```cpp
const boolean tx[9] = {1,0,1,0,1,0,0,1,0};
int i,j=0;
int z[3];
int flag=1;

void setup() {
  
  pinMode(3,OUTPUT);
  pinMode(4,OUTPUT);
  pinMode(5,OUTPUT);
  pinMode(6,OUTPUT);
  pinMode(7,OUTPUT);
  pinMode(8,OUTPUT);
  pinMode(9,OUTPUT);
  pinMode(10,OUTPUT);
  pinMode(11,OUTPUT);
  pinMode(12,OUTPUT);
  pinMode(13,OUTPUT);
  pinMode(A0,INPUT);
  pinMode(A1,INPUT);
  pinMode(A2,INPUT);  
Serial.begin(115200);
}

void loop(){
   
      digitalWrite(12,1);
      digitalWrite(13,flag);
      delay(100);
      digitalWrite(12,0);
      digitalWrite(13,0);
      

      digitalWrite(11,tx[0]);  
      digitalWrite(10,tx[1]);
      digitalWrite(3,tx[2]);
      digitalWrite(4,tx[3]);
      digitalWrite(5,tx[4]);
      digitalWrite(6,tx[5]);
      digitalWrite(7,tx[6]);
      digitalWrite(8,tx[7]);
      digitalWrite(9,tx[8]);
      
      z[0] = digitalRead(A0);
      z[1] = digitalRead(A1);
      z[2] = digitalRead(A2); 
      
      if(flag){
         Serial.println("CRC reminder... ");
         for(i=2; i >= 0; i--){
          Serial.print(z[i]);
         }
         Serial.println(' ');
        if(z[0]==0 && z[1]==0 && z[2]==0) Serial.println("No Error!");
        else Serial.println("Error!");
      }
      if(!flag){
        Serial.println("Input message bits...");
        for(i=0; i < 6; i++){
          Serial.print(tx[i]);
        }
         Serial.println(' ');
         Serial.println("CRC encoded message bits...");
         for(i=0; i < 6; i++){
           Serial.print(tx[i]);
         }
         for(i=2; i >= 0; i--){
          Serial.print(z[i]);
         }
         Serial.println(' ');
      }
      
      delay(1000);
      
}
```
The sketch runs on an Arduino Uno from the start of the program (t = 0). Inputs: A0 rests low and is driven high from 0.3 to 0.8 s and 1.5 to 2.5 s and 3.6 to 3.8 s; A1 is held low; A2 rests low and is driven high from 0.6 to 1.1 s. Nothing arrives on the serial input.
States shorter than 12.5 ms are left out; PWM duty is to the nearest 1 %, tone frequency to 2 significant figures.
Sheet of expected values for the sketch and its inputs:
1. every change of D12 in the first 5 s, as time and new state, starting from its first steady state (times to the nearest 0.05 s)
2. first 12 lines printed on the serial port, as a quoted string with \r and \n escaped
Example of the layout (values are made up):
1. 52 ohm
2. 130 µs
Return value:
1. 0 s high; 0.1 s low; 1.1 s high; 1.2 s low; 2.2 s high; 2.3 s low; 3.3 s high; 3.4 s low; 4.4 s high; 4.5 s low
2. "CRC reminder... \r\n000 \r\nNo Error!\r\nCRC reminder... \r\n000 \r\nNo Error!\r\nCRC reminder... \r\n001 \r\nError!\r\nCRC reminder... \r\n000 \r\nNo Error!\r\n"
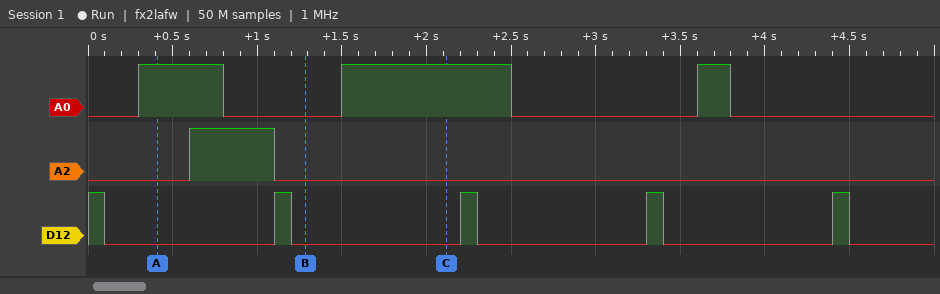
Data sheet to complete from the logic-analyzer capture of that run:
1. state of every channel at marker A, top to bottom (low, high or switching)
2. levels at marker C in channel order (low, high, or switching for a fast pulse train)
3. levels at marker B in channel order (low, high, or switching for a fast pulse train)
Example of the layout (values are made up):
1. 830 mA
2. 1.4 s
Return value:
1. A0 high, A2 low, D12 low
2. A0 high, A2 low, D12 low
3. A0 low, A2 low, D12 low
